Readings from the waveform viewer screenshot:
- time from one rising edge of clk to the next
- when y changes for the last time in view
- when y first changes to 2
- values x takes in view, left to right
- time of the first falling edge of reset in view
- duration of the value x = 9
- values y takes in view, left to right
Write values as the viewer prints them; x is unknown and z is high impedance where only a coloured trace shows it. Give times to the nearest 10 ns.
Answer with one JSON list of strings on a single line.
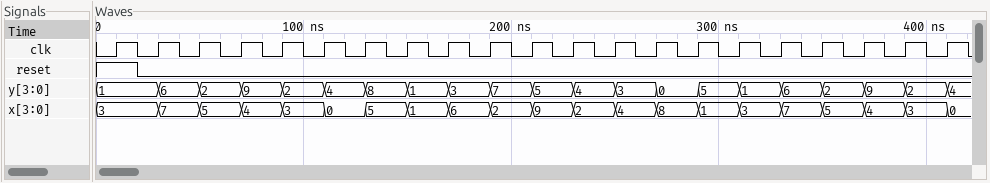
["20 ns", "410 ns", "50 ns", "3, 7, 5, 4, 3, 0, 5, 1, 6, 2, 9, 2, 4, 8, 1, 3, 7, 5, 4, 3, 0", "20 ns", "20 ns", "1, 6, 2, 9, 2, 4, 8, 1, 3, 7, 5, 4, 3, 0, 5, 1, 6, 2, 9, 2, 4"]
